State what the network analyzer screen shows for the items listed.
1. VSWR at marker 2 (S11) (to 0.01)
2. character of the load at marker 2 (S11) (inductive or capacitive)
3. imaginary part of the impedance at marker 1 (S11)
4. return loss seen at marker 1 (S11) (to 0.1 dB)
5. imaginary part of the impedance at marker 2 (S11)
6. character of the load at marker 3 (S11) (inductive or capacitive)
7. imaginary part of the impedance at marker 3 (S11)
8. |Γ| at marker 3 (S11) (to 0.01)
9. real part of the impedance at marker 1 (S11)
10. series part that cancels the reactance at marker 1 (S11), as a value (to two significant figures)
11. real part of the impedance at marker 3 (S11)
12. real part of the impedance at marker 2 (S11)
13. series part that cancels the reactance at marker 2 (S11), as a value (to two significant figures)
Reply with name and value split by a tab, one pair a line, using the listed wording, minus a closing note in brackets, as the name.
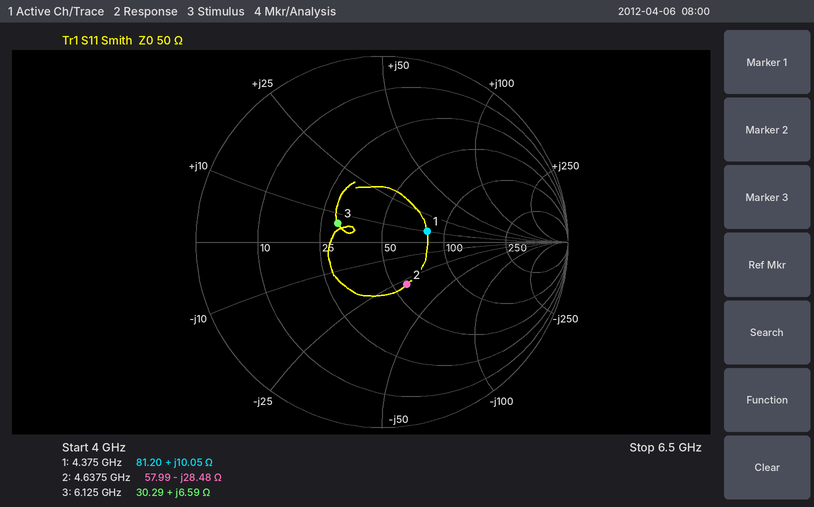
VSWR at marker 2 (S11)	1.72
character of the load at marker 2 (S11)	capacitive
imaginary part of the impedance at marker 1	+10.05 Ω
return loss seen at marker 1 (S11)	12.1 dB
imaginary part of the impedance at marker 2	-28.48 Ω
character of the load at marker 3 (S11)	inductive
imaginary part of the impedance at marker 3	+6.59 Ω
|Γ| at marker 3 (S11)	0.26
real part of the impedance at marker 1	81.20 Ω
series part that cancels the reactance at marker 1 (S11), as a value	3.6 pF
real part of the impedance at marker 3	30.29 Ω
real part of the impedance at marker 2	57.99 Ω
series part that cancels the reactance at marker 2 (S11), as a value	980 pH
